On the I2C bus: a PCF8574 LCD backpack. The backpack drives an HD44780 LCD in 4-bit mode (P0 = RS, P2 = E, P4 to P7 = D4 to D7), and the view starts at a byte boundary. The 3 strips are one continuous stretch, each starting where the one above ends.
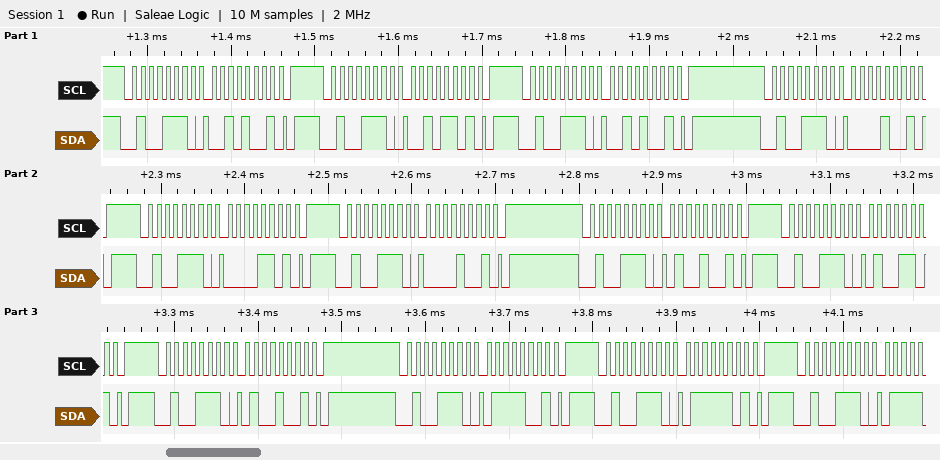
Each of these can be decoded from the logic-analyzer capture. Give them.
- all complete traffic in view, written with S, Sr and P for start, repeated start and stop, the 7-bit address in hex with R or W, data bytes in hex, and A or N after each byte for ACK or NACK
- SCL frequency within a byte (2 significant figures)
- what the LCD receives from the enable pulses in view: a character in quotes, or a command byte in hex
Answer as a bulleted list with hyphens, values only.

- S 27W A 29 A P S 27W A 2D A P S 27W A 29 A P S 27W A 09 A P S 27W A 0D A P S 27W A 09 A P S 27W A 49 A P S 27W A 4D A P S 27W A 49 A P S 27W A 79 A P S 27W A 7D A P S 27W A
- 100 kHz
- ' '
